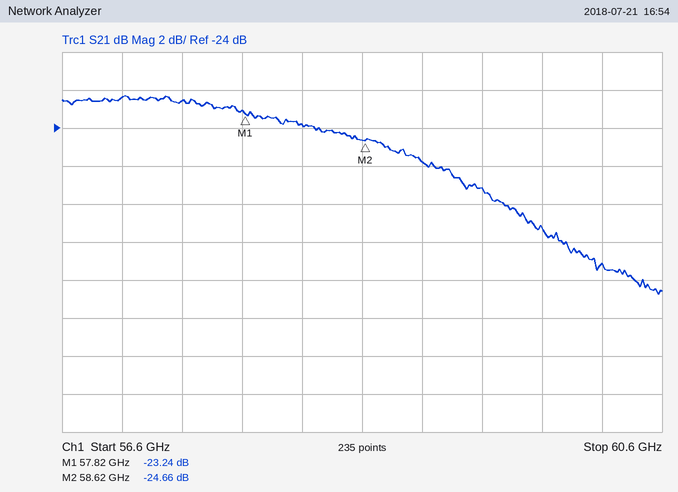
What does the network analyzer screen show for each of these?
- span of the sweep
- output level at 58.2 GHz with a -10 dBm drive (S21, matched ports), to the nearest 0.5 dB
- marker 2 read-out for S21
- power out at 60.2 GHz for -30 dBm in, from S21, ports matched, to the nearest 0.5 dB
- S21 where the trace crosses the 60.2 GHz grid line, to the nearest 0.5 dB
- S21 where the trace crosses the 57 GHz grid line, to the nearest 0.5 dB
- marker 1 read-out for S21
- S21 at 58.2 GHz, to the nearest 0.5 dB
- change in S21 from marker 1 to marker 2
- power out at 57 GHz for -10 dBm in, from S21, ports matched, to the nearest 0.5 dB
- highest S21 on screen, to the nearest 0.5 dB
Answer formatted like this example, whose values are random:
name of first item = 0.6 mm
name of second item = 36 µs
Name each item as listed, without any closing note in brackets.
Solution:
span of the sweep = 4 GHz
output level at 58.2 GHz with a -10 dBm drive (S21, matched ports), to the nearest 0.5 dB = -34.0 dBm
marker 2 read-out for S21 = -24.66 dB
power out at 60.2 GHz for -30 dBm in, from S21, ports matched, to the nearest 0.5 dB = -61.0 dBm
S21 where the trace crosses the 60.2 GHz grid line, to the nearest 0.5 dB = -31.0 dB
S21 where the trace crosses the 57 GHz grid line, to the nearest 0.5 dB = -22.5 dB
marker 1 read-out for S21 = -23.24 dB
S21 at 58.2 GHz, to the nearest 0.5 dB = -24.0 dB
change in S21 from marker 1 to marker 2 = -1.42 dB
power out at 57 GHz for -10 dBm in, from S21, ports matched, to the nearest 0.5 dB = -32.5 dBm
highest S21 on screen, to the nearest 0.5 dB = -22.5 dB
